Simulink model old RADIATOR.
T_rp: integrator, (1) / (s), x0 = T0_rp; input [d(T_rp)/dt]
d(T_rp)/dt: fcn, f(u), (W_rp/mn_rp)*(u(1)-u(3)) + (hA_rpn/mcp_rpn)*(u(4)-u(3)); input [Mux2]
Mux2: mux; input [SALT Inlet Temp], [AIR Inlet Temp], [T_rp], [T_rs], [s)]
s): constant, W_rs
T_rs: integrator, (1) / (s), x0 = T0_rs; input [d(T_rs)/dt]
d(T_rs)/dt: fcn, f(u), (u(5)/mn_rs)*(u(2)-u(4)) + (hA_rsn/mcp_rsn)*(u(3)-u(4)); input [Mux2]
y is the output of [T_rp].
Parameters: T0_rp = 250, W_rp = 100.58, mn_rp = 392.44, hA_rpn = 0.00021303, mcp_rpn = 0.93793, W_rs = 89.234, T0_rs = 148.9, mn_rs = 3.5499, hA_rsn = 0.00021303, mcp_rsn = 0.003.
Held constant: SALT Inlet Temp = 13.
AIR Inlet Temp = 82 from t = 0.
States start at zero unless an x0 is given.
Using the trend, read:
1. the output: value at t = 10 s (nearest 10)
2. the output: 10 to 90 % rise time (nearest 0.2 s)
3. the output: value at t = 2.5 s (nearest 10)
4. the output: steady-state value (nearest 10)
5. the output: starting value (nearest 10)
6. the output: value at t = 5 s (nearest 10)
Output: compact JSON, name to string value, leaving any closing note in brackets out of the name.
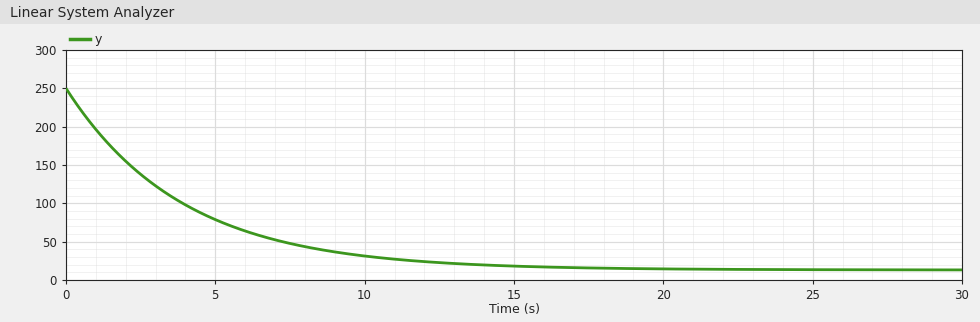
{"the output: value at t = 10 s": "30", "the output: 10 to 90 % rise time": "8.6 s", "the output: value at t = 2.5 s": "140", "the output: steady-state value": "10", "the output: starting value": "250", "the output: value at t = 5 s": "80"}
